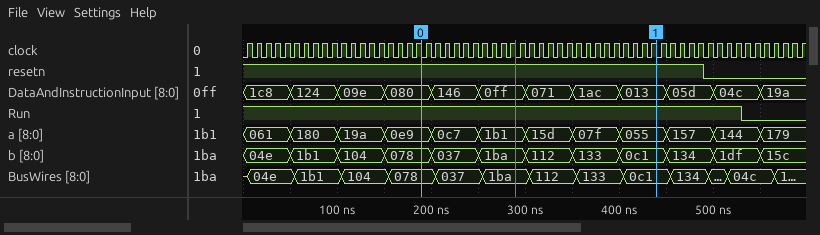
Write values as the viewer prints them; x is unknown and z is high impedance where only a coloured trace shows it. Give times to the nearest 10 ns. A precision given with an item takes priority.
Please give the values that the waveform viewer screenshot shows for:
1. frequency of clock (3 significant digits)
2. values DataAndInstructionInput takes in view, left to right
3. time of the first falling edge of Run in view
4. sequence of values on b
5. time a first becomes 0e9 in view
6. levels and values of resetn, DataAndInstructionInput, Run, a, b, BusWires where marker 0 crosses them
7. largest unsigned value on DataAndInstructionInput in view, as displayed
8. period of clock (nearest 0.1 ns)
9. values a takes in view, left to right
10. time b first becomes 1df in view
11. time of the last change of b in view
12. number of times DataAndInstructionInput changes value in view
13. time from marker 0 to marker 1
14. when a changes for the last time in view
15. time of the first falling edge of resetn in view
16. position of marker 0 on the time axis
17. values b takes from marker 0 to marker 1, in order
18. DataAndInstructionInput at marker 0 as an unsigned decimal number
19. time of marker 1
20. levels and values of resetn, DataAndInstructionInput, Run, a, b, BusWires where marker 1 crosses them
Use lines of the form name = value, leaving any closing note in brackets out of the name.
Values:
frequency of clock = 100 MHz
values DataAndInstructionInput takes in view, left to right = 1c8, 124, 09e, 080, 146, 0ff, 071, 1ac, 013, 05d, 04c, 19a
time of the first falling edge of Run in view = 530 ns
sequence of values on b = 04e, 1b1, 104, 078, 037, 1ba, 112, 133, 0c1, 134, 1df, 15c
time a first becomes 0e9 in view = 150 ns
levels and values of resetn, DataAndInstructionInput, Run, a, b, BusWires where marker 0 crosses them = resetn=1, DataAndInstructionInput=080, Run=1, a=0e9, b=078, BusWires=078
largest unsigned value on DataAndInstructionInput in view, as displayed = 1c8
period of clock = 10 ns
values a takes in view, left to right = 061, 180, 19a, 0e9, 0c7, 1b1, 15d, 07f, 055, 157, 144, 179
time b first becomes 1df in view = 500 ns
time of the last change of b in view = 550 ns
number of times DataAndInstructionInput changes value in view = 11
time from marker 0 to marker 1 = 250 ns
when a changes for the last time in view = 550 ns
time of the first falling edge of resetn in view = 490 ns
position of marker 0 on the time axis = 190 ns
values b takes from marker 0 to marker 1, in order = 078, 037, 1ba, 112, 133, 0c1
DataAndInstructionInput at marker 0 as an unsigned decimal number = 128
time of marker 1 = 440 ns
levels and values of resetn, DataAndInstructionInput, Run, a, b, BusWires where marker 1 crosses them = resetn=1, DataAndInstructionInput=013, Run=1, a=055, b=0c1, BusWires=0c1
